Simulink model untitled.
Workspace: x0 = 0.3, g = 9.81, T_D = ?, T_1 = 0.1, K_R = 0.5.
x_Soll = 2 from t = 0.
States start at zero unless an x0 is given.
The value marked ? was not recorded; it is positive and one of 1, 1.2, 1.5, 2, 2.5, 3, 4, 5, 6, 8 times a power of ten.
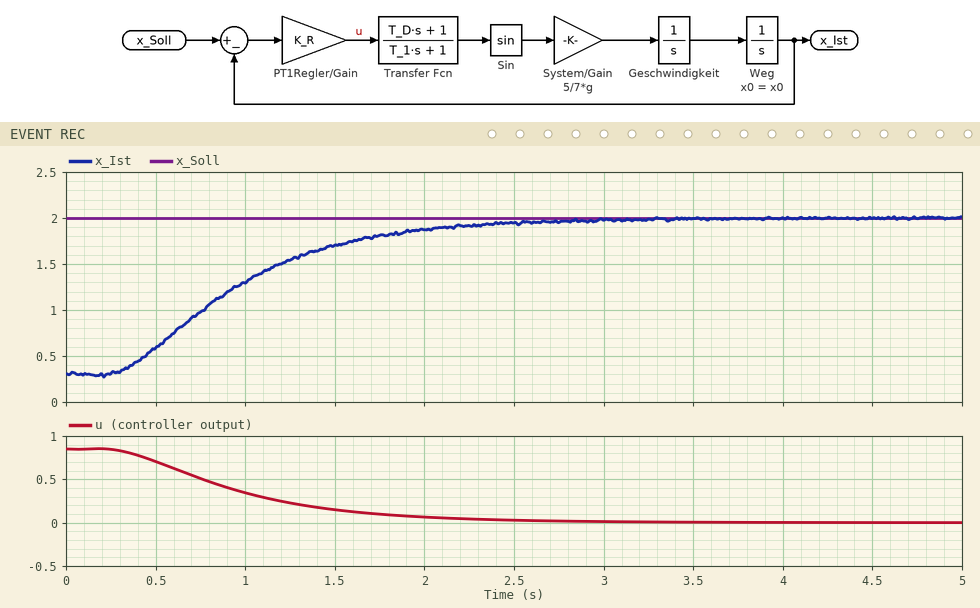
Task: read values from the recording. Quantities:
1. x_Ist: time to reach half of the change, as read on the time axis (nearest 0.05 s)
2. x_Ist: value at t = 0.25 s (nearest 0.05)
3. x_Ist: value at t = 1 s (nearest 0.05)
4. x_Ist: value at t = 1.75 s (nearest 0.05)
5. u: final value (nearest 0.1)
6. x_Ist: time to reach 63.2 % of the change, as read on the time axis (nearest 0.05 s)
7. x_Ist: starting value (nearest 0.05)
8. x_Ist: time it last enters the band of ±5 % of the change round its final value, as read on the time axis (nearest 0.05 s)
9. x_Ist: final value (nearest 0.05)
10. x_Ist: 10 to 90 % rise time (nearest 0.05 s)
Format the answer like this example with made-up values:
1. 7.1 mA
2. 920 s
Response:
1. 0.85 s
2. 0.30
3. 1.30
4. 1.80
5. 0.0
6. 1.05 s
7. 0.30
8. 2.25 s
9. 2.00
10. 1.40 s
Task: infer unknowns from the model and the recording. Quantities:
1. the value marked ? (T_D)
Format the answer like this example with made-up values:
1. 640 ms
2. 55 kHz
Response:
1. 1
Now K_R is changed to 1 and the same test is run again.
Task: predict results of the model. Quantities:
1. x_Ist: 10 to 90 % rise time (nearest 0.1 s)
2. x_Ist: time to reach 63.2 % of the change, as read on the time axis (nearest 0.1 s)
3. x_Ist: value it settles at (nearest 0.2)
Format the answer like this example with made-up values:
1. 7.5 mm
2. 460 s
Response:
1. 1.8 s
2. 1.3 s
3. 2.0
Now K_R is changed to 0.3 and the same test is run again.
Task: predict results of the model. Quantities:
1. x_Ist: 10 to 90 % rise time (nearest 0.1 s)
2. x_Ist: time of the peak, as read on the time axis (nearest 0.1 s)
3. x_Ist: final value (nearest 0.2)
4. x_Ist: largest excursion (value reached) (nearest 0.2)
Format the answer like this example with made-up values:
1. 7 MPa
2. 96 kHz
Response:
1. 1.2 s
2. 2.6 s
3. 2.0
4. 2.0
